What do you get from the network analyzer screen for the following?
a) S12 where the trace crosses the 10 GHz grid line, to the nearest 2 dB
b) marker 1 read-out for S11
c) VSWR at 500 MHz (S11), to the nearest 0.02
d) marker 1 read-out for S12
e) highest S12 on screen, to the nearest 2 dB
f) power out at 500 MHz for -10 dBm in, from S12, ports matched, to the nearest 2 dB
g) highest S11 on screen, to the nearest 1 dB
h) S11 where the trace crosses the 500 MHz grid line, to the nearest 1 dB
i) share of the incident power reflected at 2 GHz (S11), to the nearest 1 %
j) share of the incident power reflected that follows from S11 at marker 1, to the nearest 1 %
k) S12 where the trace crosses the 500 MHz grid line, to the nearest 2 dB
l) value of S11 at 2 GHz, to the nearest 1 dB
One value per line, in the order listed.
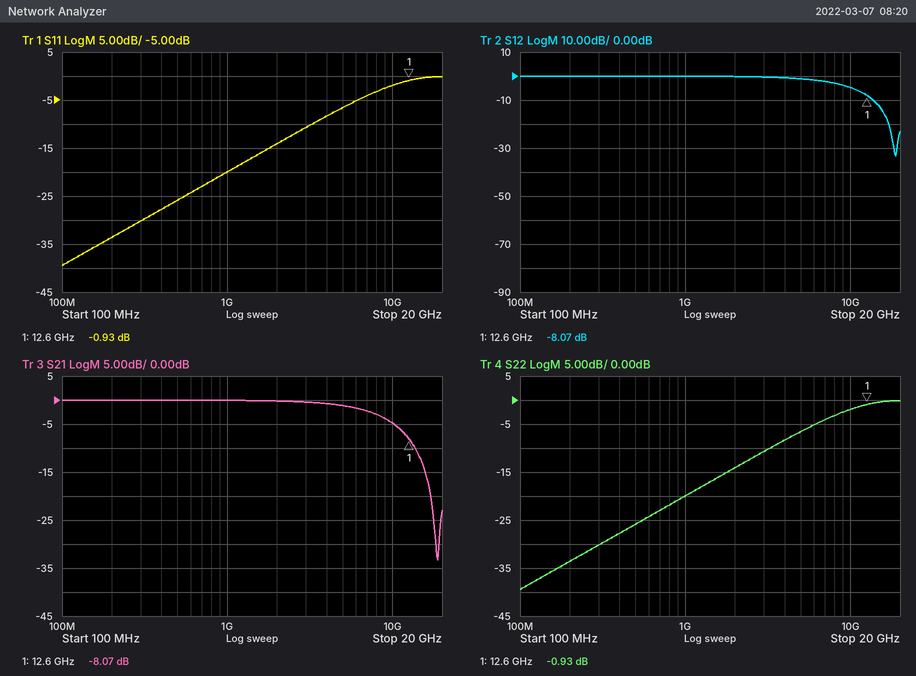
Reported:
-4 dB
-0.93 dB
1.10
-8.07 dB
0 dB
-10 dBm
0 dB
-26 dB
4 %
81 %
0 dB
-14 dB
